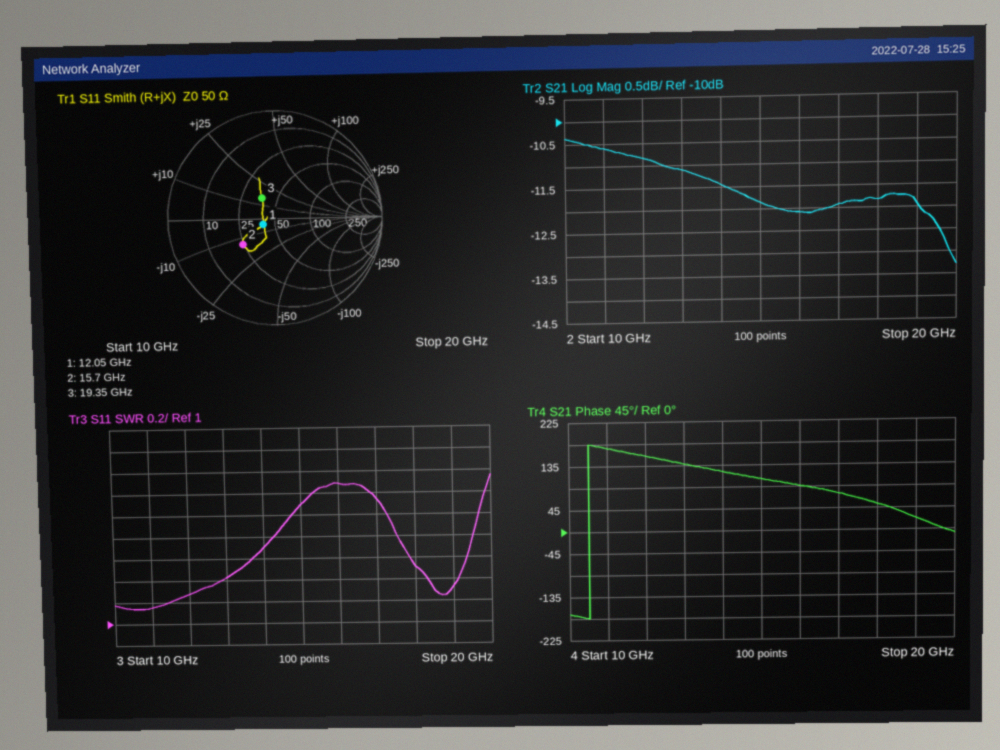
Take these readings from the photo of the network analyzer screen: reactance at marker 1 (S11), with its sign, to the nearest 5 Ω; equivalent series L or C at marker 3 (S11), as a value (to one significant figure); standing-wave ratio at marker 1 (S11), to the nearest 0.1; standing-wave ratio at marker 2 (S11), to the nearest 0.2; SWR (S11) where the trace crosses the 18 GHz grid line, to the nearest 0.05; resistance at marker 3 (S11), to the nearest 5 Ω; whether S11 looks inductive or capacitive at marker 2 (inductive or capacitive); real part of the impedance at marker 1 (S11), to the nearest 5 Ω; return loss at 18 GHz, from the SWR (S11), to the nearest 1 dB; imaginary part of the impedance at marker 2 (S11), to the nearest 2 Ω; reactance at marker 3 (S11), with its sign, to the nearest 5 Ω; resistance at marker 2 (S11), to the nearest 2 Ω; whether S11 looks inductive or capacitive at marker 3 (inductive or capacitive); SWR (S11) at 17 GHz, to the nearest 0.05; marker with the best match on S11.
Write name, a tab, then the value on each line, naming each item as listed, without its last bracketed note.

reactance at marker 1 (S11), with its sign, to the nearest 5 Ω	-5 Ω
equivalent series L or C at marker 3 (S11), as a value	100 pH
standing-wave ratio at marker 1 (S11), to the nearest 0.1	1.3
standing-wave ratio at marker 2 (S11), to the nearest 0.2	2.2
SWR (S11) where the trace crosses the 18 GHz grid line, to the nearest 0.05	1.50
resistance at marker 3 (S11), to the nearest 5 Ω	35 Ω
whether S11 looks inductive or capacitive at marker 2	capacitive
real part of the impedance at marker 1 (S11), to the nearest 5 Ω	40 Ω
return loss at 18 GHz, from the SWR (S11), to the nearest 1 dB	14 dB
imaginary part of the impedance at marker 2 (S11), to the nearest 2 Ω	-14 Ω
reactance at marker 3 (S11), with its sign, to the nearest 5 Ω	+15 Ω
resistance at marker 2 (S11), to the nearest 2 Ω	24 Ω
whether S11 looks inductive or capacitive at marker 3	inductive
SWR (S11) at 17 GHz, to the nearest 0.05	2.15
marker with the best match on S11	marker 1
